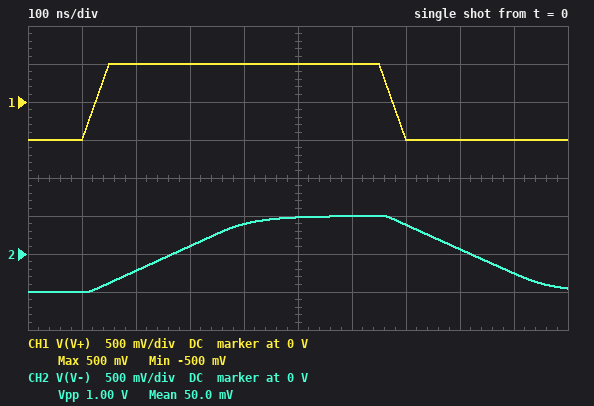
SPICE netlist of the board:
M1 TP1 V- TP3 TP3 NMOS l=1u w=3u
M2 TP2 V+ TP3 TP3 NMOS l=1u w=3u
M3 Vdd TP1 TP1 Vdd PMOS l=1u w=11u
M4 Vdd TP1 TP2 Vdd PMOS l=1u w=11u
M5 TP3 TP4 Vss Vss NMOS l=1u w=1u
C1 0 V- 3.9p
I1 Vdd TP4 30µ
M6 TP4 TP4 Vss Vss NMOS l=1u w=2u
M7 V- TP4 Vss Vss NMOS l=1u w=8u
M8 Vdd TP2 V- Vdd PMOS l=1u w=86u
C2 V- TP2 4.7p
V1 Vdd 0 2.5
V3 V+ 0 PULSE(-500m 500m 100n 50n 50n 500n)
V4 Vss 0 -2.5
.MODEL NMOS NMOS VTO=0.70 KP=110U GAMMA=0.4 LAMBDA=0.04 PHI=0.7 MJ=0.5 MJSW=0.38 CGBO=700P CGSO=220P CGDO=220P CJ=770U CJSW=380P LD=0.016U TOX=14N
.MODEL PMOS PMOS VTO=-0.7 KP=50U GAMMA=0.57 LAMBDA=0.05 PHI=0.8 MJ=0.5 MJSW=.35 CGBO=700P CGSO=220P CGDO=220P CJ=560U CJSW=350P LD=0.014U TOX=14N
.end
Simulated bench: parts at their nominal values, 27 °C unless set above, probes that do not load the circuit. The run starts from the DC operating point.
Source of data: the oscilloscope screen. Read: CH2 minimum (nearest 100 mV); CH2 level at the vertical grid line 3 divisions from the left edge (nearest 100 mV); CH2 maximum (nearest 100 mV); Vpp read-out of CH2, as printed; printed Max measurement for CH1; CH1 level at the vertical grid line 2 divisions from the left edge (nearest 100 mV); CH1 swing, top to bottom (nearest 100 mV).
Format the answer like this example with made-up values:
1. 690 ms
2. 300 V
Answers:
1. -500 mV
2. 100 mV
3. 500 mV
4. 1.00 V
5. 500 mV
6. 500 mV
7. 1.0 V
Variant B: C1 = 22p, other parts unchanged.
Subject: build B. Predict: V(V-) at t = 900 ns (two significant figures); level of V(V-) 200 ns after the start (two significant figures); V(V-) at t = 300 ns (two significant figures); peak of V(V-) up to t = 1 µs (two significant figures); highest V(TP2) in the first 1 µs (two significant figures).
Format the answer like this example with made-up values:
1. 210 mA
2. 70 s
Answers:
1. -180 mV
2. -270 mV
3. 58 mV
4. 500 mV
5. 1.7 V
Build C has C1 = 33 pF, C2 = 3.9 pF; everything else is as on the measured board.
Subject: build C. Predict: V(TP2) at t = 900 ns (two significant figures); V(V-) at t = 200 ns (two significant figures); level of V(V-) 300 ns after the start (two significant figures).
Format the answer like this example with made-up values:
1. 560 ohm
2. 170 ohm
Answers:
1. 1.8 V
2. -240 mV
3. 150 mV
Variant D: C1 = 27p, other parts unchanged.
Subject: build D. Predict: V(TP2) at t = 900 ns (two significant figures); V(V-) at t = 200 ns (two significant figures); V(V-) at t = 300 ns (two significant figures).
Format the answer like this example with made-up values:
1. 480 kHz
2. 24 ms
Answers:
1. 1.7 V
2. -280 mV
3. 47 mV
